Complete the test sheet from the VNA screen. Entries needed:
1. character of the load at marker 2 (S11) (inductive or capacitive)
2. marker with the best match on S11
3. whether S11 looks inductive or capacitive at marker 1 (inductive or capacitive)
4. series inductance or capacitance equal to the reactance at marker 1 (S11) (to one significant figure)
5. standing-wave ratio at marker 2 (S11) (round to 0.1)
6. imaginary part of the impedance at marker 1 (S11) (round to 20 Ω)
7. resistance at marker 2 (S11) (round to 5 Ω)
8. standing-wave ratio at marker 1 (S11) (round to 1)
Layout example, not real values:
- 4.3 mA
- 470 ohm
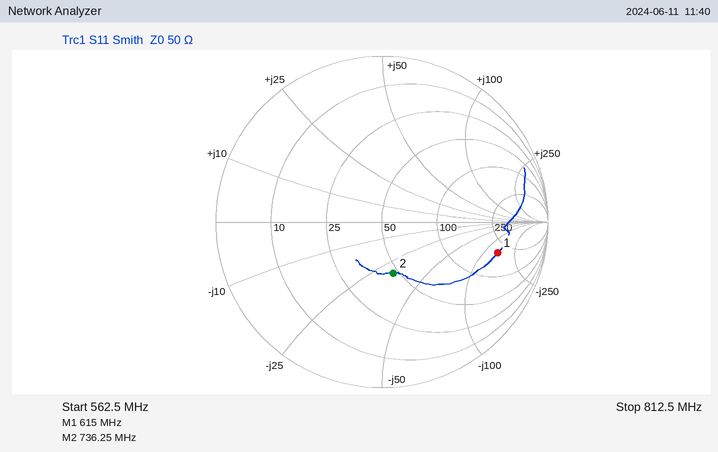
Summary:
- capacitive
- marker 2
- capacitive
- 2 pF
- 1.9
- -140 Ω
- 45 Ω
- 6
